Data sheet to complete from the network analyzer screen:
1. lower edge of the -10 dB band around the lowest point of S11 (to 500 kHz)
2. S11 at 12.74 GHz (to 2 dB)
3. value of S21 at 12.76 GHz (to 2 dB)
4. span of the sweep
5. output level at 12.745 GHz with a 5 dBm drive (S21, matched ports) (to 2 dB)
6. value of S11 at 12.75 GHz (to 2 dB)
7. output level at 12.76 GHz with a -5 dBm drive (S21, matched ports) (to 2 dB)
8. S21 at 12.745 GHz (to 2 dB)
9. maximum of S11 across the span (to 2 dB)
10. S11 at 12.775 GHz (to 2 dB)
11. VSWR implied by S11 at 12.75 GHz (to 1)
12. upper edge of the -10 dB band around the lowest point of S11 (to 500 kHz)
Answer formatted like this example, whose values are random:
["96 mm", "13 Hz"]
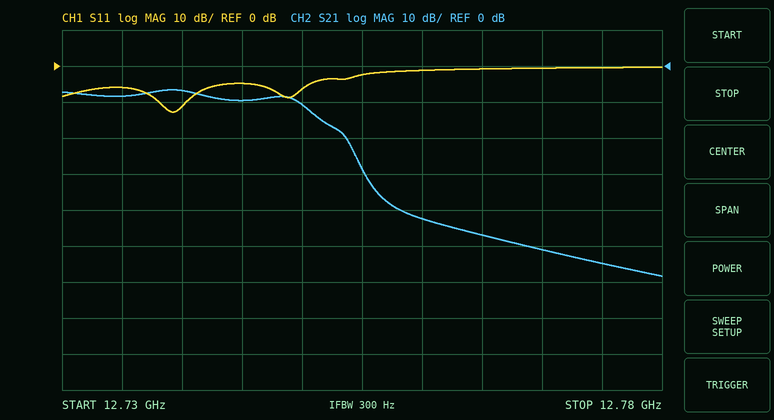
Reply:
["12.7380 GHz", "-12 dB", "-42 dB", "50 MHz", "-4 dBm", "-6 dB", "-48 dBm", "-10 dB", "0 dB", "0 dB", "3", "12.7405 GHz"]
